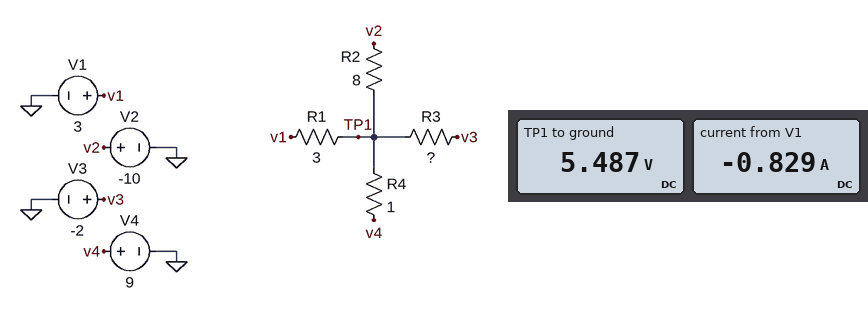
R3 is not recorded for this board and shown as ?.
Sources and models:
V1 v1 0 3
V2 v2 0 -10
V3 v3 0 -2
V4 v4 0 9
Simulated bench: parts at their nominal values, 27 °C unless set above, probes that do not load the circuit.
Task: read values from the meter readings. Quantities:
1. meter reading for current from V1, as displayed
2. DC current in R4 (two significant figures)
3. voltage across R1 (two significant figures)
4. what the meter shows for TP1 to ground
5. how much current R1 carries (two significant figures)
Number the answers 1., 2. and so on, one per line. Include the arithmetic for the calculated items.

1. -0.829 A
2. (9 V - 5.487 V) / 1 Ω = 3.5 A
3. 5.487 V - 3 V = 2.5 V
4. 5.487 V
5. (5.487 V - 3 V) / 3 Ω = 830 mA
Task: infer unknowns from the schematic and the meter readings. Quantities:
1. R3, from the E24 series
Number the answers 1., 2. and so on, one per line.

1. 10 Ω
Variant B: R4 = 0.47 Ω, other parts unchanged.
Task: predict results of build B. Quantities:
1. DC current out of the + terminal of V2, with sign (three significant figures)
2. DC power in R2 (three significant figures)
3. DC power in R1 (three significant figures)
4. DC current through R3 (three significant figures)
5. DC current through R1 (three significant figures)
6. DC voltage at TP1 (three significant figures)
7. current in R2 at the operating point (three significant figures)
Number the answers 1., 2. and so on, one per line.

1. -2.12 A
2. 36.0 W
3. 5.23 W
4. 896 mA
5. 1.32 A
6. 6.96 V
7. 2.12 A
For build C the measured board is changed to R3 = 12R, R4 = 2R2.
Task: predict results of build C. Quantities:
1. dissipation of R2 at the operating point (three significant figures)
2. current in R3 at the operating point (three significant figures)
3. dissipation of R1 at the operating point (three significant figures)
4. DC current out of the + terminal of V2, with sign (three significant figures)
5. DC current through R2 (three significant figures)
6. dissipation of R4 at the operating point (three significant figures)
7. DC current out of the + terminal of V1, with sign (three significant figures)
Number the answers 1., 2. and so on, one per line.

1. 23.4 W
2. 474 mA
3. 158 mW
4. -1.71 A
5. 1.71 A
6. 12.8 W
7. -229 mA
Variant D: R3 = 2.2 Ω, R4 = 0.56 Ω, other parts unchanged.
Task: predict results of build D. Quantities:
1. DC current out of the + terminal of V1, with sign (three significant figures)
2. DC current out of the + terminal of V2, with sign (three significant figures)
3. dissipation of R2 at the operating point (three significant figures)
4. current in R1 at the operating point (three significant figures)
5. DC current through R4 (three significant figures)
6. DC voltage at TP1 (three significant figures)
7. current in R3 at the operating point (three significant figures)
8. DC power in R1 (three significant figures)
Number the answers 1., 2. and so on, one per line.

1. -842 mA
2. -1.94 A
3. 30.1 W
4. 842 mA
5. 6.20 A
6. 5.53 V
7. 3.42 A
8. 2.13 W
